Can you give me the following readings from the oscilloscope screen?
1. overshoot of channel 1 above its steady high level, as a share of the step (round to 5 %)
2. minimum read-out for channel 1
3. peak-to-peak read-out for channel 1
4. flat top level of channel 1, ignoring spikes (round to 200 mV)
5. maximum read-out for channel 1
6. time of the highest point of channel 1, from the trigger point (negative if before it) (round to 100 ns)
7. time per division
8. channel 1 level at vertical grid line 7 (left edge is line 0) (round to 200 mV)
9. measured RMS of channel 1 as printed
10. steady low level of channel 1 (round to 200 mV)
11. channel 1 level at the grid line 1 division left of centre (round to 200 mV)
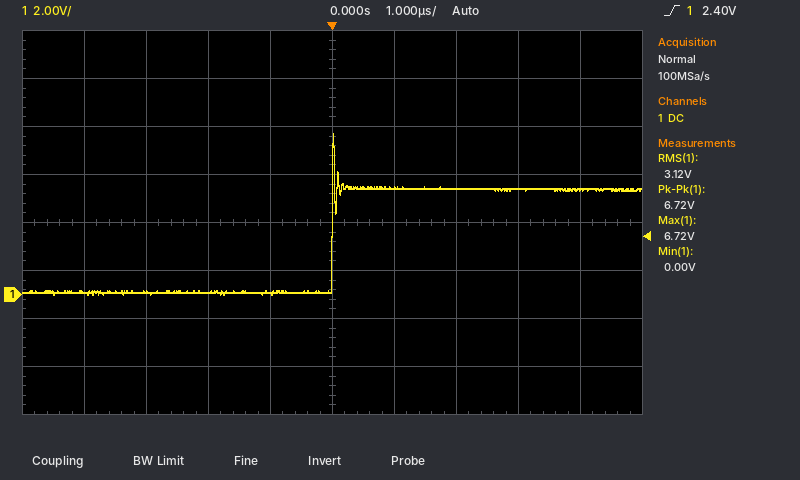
55 %
0.00 V
6.72 V
4.4 V
6.72 V
0.0 µs
1 µs
4.4 V
3.12 V
0.0 V
0.0 V
